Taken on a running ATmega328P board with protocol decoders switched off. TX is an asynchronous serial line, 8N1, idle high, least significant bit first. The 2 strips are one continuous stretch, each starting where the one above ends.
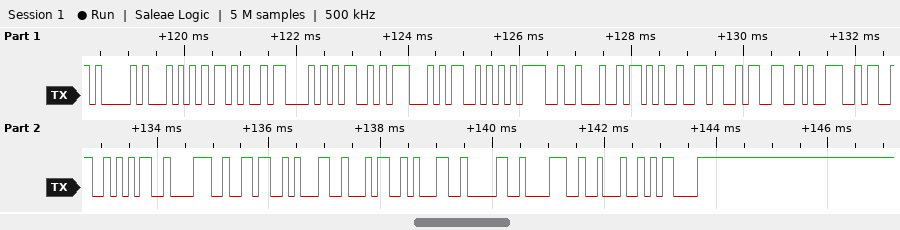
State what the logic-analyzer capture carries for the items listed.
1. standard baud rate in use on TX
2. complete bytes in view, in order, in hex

9600 baud
0x41 0x54 0x2B 0x43 0x4D 0x47 0x53 0x3D 0x22 0x2B 0x36 0x33 0x39 0x33 0x35 0x38 0x36 0x31 0x34 0x31 0x30 0x38 0x22 0x0D
